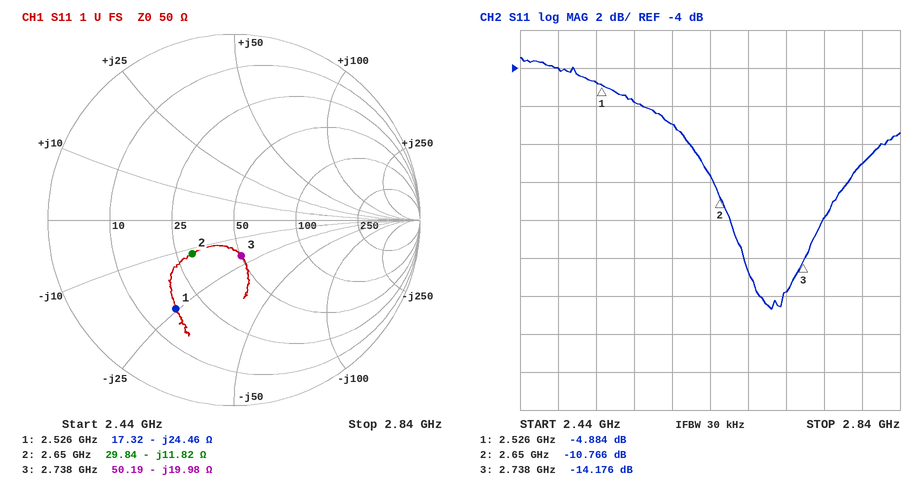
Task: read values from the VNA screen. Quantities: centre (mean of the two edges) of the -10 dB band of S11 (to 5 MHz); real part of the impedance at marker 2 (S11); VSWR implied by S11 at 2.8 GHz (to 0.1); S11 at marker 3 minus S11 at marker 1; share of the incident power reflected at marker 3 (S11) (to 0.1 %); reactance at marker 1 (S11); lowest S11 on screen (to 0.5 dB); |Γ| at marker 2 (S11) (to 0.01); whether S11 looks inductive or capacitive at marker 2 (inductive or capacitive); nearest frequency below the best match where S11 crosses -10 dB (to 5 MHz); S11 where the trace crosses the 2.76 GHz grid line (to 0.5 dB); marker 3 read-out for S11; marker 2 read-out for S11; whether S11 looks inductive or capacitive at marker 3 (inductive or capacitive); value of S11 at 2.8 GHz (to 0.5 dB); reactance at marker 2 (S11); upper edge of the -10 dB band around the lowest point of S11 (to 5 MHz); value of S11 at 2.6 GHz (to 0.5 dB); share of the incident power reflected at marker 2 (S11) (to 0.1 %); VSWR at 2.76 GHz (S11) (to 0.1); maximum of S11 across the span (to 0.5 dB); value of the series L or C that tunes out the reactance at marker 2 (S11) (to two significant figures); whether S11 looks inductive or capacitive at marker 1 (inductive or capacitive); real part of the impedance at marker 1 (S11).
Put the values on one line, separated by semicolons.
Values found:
2.715 GHz; 29.84 Ω; 2.1; -9.292 dB; 3.8 %; -24.46 Ω; -16.5 dB; 0.29; capacitive; 2.645 GHz; -12.0 dB; -14.176 dB; -10.766 dB; capacitive; -9.0 dB; -11.82 Ω; 2.785 GHz; -7.0 dB; 8.4 %; 1.7; -3.5 dB; 710 pH; capacitive; 17.32 Ω
